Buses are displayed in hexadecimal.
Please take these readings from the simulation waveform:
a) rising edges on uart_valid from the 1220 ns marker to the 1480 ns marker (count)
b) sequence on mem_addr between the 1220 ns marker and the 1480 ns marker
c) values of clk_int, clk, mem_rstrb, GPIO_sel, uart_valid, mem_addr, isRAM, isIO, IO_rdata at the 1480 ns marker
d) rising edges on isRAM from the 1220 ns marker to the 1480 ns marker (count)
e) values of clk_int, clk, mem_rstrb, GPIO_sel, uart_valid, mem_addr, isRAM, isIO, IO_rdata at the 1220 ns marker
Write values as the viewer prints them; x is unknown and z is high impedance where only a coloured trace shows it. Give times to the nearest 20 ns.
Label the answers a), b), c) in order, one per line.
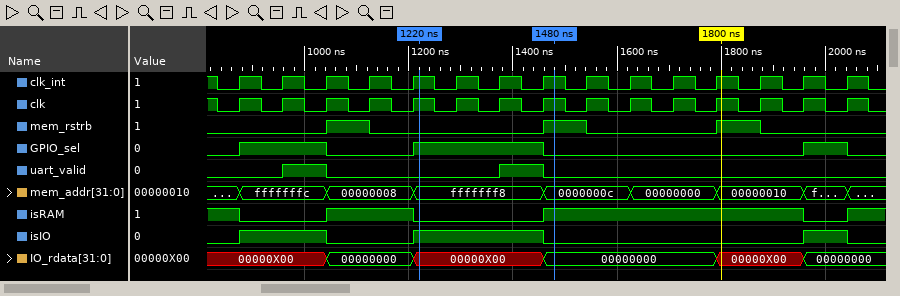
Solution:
a) 1
b) fffffff8, 0000000c
c) clk_int=1, clk=1, mem_rstrb=1, GPIO_sel=0, uart_valid=0, mem_addr=0000000c, isRAM=1, isIO=0, IO_rdata=00000000
d) 1
e) clk_int=1, clk=1, mem_rstrb=0, GPIO_sel=1, uart_valid=0, mem_addr=fffffff8, isRAM=0, isIO=1, IO_rdata=00000X00
